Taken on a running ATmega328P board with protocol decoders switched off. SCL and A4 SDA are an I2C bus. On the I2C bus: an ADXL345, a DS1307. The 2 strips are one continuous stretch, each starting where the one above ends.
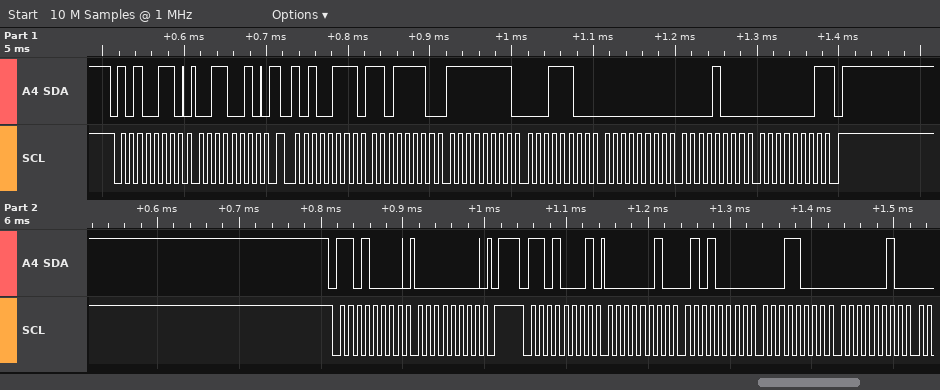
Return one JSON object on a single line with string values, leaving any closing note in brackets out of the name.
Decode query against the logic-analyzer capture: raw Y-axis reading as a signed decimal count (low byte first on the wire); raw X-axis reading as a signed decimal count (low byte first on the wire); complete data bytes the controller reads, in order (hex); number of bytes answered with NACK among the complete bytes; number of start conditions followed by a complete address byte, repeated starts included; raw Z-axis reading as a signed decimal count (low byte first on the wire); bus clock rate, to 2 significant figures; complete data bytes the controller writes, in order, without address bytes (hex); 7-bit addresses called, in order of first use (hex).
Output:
{"raw Y-axis reading as a signed decimal count": "28", "raw X-axis reading as a signed decimal count": "-34", "complete data bytes the controller reads, in order": "DE FF 1C 00 08 01 02 50 18 02", "number of bytes answered with NACK among the complete bytes": "1", "number of start conditions followed by a complete address byte, repeated starts included": "4", "raw Z-axis reading as a signed decimal count": "264", "bus clock rate, to 2 significant figures": "100 kHz", "complete data bytes the controller writes, in order, without address bytes": "32 00", "7-bit addresses called, in order of first use": "0x53 0x68"}
